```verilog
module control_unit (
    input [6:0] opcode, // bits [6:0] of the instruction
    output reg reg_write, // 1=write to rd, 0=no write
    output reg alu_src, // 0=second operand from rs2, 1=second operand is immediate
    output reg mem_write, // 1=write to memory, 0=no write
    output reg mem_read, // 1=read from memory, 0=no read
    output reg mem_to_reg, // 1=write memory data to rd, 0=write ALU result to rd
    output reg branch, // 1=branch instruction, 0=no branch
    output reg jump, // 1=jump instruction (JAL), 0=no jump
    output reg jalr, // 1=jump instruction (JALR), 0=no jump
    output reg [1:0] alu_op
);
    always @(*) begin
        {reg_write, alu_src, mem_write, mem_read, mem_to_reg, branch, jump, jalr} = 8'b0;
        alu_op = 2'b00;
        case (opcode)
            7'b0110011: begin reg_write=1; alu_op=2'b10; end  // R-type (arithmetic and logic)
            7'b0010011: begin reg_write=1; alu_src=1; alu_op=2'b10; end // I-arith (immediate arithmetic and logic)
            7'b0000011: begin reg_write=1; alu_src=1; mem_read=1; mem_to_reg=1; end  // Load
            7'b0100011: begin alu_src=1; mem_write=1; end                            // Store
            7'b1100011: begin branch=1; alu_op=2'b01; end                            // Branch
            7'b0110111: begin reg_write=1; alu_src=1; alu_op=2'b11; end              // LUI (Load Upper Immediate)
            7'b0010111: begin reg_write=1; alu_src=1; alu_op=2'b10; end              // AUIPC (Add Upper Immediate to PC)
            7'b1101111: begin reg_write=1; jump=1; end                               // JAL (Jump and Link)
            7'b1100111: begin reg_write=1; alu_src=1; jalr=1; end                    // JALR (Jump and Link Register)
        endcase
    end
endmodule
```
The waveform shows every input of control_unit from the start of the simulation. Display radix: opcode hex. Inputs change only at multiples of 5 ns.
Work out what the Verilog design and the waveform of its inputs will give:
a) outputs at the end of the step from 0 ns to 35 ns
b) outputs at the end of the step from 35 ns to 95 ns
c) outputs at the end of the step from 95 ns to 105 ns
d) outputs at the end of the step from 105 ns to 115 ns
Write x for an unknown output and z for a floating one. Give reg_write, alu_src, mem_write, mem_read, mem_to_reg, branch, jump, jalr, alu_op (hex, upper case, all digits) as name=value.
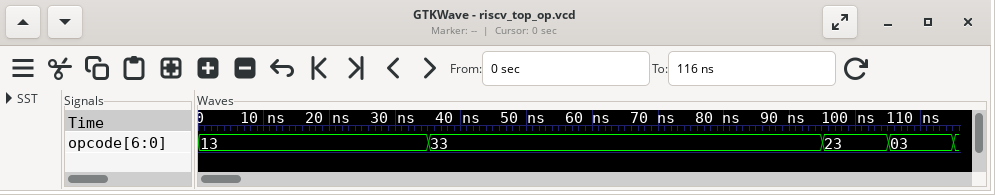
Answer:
reg_write=1, alu_src=1, mem_write=0, mem_read=0, mem_to_reg=0, branch=0, jump=0, jalr=0, alu_op=2
reg_write=1, alu_src=0, mem_write=0, mem_read=0, mem_to_reg=0, branch=0, jump=0, jalr=0, alu_op=2
reg_write=0, alu_src=1, mem_write=1, mem_read=0, mem_to_reg=0, branch=0, jump=0, jalr=0, alu_op=0
reg_write=1, alu_src=1, mem_write=0, mem_read=1, mem_to_reg=1, branch=0, jump=0, jalr=0, alu_op=0
